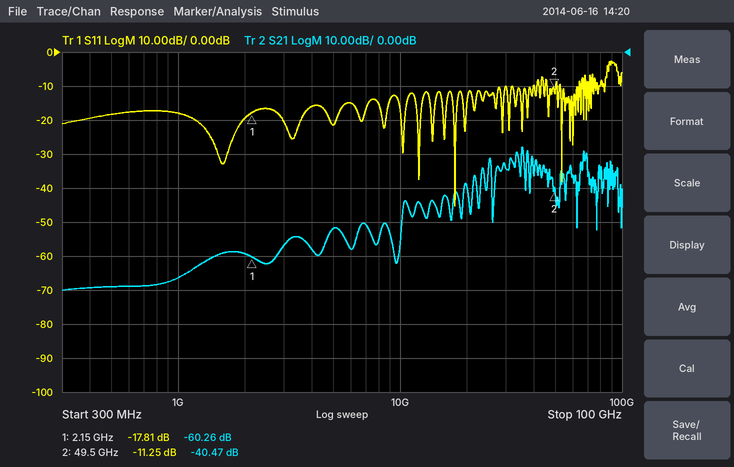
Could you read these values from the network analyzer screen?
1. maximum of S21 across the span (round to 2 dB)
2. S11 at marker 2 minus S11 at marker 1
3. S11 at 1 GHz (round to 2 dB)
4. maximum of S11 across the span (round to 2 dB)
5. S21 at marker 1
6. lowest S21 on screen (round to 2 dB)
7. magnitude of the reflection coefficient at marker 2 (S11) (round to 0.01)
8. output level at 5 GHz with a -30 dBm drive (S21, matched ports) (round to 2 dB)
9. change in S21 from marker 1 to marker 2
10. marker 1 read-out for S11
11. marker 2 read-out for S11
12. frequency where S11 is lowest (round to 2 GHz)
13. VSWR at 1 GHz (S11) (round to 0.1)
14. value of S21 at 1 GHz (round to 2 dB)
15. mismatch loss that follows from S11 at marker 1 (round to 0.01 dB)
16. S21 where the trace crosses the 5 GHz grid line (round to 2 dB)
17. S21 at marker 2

-28 dB
6.56 dB
-18 dB
-2 dB
-60.26 dB
-70 dB
0.27
-82 dBm
19.79 dB
-17.81 dB
-11.25 dB
18 GHz
1.3
-66 dB
0.07 dB
-52 dB
-40.47 dB
